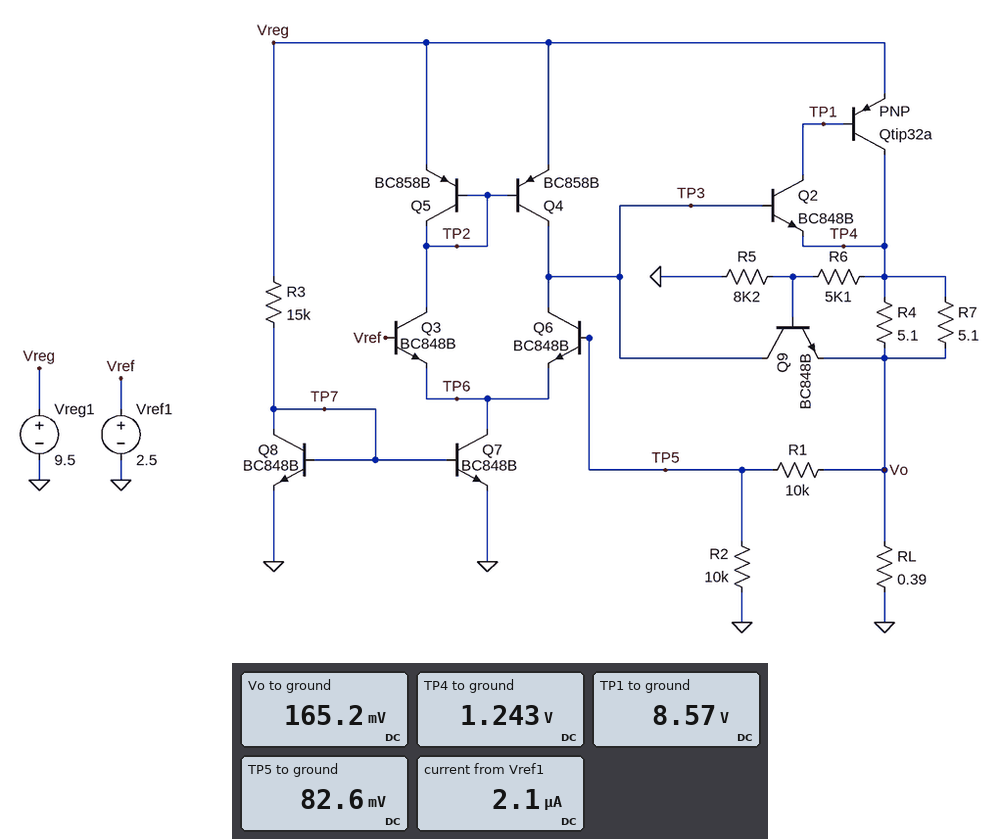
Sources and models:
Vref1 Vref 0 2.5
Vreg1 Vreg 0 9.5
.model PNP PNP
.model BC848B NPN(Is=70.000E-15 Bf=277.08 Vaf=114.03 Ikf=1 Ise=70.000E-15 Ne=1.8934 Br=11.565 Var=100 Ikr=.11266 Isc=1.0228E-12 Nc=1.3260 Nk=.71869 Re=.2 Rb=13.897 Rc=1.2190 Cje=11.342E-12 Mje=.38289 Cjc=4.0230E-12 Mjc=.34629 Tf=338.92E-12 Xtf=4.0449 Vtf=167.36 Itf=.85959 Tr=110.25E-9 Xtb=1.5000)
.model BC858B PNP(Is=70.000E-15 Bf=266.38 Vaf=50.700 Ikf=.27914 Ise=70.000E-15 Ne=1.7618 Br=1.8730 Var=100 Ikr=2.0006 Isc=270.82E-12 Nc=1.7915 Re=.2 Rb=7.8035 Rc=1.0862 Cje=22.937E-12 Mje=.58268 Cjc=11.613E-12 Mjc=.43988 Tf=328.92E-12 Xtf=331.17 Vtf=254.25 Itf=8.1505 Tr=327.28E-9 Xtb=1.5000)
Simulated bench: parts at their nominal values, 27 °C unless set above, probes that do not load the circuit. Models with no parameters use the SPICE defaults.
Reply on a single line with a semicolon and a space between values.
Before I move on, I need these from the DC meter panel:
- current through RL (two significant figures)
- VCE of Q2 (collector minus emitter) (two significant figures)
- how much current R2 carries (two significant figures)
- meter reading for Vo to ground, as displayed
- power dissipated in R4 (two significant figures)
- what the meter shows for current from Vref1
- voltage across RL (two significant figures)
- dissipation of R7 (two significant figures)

420 mA; 7.3 V; 8.3 µA; 165.2 mV; 230 mW; 2.1 µA; 170 mV; 230 mW
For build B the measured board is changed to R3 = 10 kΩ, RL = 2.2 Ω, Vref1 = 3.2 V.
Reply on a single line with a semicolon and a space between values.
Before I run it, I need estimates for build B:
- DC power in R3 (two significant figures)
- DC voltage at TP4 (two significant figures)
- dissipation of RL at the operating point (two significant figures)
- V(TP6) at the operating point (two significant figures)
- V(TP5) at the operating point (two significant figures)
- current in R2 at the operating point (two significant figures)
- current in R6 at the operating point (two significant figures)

7.9 mW; 4.0 V; 1.6 W; 2.6 V; 930 mV; 93 µA; 300 µA
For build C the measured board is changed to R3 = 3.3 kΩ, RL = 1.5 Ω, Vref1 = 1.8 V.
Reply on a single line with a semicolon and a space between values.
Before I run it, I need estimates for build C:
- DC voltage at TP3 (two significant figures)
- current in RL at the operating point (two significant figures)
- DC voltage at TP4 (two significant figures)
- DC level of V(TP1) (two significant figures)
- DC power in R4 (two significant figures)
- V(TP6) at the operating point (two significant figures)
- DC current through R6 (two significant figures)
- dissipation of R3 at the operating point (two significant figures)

3.4 V; 670 mA; 2.7 V; 8.6 V; 570 mW; 1.2 V; 210 µA; 24 mW
